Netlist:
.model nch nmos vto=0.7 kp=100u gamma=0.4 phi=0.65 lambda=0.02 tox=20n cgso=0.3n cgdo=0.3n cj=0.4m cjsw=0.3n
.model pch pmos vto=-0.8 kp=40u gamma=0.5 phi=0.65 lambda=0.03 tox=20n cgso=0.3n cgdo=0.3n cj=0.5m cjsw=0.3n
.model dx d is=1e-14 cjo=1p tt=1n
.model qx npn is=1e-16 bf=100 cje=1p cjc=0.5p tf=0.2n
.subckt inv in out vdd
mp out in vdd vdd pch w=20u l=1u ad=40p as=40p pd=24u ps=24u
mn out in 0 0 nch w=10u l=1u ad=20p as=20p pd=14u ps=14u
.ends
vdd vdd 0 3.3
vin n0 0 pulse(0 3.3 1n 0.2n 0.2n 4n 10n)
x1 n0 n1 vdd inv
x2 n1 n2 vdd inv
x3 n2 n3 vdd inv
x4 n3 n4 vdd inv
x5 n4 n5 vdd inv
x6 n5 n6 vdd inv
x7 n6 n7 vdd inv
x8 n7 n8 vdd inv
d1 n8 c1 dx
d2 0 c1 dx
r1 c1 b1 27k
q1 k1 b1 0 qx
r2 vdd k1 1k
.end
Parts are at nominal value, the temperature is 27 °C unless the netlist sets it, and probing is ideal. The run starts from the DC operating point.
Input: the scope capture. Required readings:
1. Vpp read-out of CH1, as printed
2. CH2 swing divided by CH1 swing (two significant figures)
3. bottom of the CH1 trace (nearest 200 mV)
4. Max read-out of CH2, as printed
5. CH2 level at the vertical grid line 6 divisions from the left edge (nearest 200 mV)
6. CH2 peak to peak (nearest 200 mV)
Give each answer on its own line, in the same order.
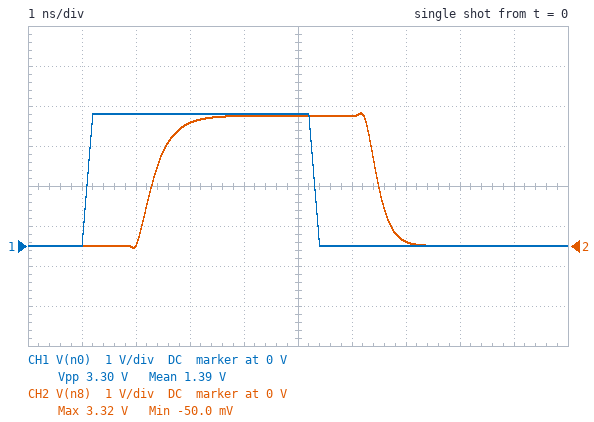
3.30 V
1.0
0 V
3.32 V
3.2 V
3.4 V
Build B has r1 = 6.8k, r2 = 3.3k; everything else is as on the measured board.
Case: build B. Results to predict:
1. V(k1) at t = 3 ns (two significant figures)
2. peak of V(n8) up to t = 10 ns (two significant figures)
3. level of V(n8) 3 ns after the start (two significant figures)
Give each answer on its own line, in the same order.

3.4 V
3.2 V
3.0 V
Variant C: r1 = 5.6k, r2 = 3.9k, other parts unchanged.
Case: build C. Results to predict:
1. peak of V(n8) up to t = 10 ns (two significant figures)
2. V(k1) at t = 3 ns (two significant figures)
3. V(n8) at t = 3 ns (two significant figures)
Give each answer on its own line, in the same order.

3.2 V
3.4 V
3.0 V
